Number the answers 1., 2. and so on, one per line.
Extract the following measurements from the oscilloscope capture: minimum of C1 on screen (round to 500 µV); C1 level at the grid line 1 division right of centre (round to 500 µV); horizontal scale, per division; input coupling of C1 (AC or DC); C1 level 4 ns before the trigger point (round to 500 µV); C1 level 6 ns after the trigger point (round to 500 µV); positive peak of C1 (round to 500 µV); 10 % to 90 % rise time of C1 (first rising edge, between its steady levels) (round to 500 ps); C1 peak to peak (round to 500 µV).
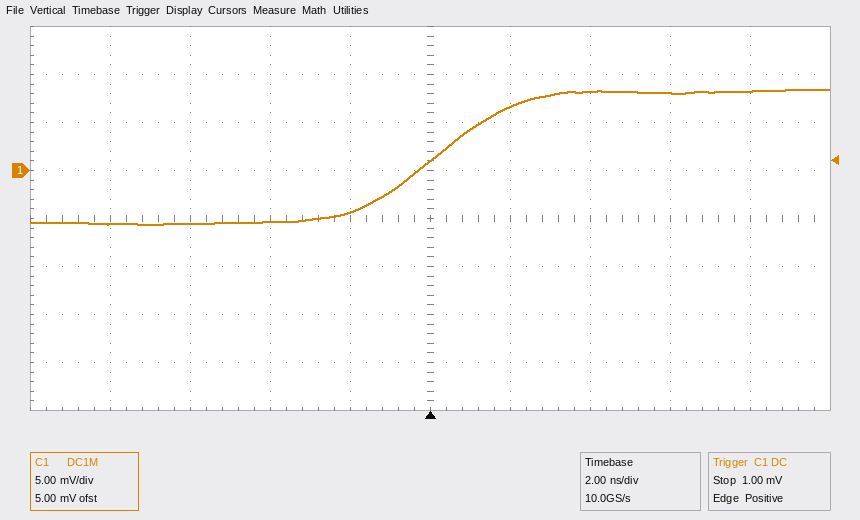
1. -5.5 mV
2. 6.5 mV
3. 2 ns
4. DC
5. -5.5 mV
6. 8.0 mV
7. 8.5 mV
8. 4.0 ns
9. 14.0 mV
